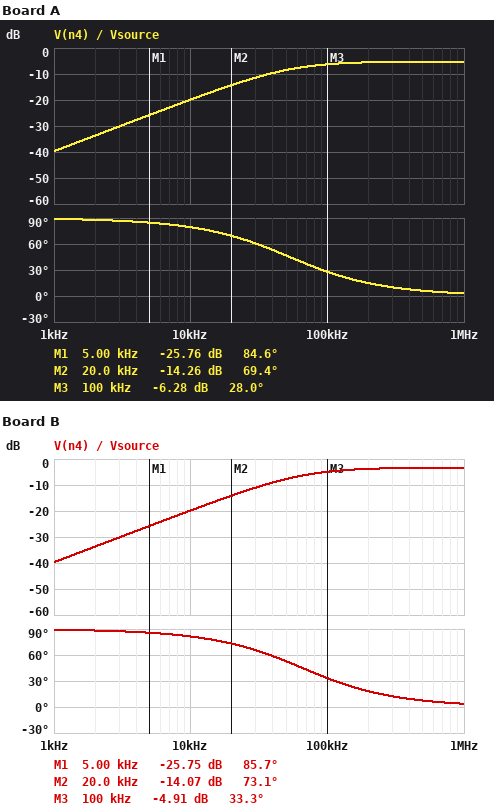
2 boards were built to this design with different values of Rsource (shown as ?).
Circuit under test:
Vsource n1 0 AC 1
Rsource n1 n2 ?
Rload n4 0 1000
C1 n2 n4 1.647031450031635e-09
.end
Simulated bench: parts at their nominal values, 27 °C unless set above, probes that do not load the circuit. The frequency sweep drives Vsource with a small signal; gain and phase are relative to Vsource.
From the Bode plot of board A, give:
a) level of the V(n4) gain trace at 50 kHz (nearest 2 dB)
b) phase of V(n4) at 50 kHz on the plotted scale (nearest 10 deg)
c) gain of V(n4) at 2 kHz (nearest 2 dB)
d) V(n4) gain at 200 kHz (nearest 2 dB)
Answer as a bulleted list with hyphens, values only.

- -8 dB
- 50 deg
- -34 dB
- -6 dB
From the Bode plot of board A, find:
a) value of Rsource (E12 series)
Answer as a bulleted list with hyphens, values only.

- 820 Ω
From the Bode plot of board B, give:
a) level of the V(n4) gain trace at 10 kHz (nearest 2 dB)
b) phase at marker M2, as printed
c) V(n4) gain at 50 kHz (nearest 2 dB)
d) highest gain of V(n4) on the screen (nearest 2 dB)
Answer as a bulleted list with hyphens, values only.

- -20 dB
- 73.1 deg
- -8 dB
- -4 dB
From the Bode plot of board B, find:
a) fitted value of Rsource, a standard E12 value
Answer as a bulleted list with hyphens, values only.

- 470 Ω
